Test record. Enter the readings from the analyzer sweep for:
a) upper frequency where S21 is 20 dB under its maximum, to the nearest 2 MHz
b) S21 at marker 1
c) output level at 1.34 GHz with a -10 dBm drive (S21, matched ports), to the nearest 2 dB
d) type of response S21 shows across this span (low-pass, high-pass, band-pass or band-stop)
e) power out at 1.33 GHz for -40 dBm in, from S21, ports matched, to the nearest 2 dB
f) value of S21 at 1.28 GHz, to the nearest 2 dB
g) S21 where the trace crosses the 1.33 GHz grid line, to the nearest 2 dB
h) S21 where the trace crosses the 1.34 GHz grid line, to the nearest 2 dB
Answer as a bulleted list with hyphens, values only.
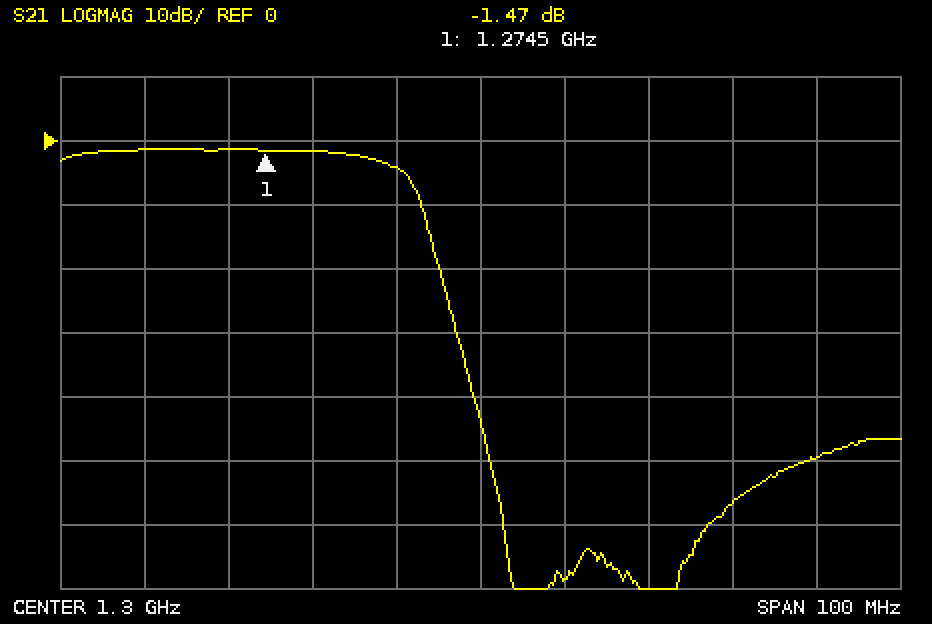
- 1.296 GHz
- -1.47 dB
- -60 dBm
- low-pass
- -96 dBm
- -2 dB
- -56 dB
- -50 dB
